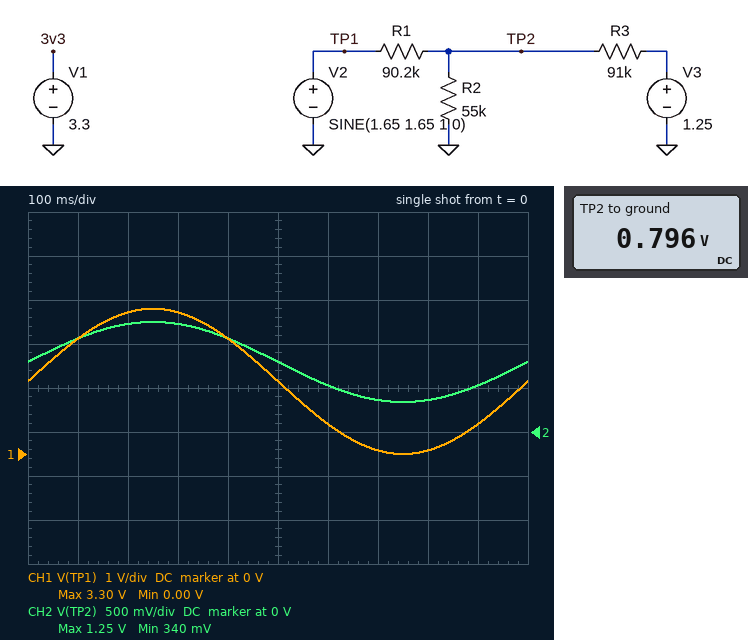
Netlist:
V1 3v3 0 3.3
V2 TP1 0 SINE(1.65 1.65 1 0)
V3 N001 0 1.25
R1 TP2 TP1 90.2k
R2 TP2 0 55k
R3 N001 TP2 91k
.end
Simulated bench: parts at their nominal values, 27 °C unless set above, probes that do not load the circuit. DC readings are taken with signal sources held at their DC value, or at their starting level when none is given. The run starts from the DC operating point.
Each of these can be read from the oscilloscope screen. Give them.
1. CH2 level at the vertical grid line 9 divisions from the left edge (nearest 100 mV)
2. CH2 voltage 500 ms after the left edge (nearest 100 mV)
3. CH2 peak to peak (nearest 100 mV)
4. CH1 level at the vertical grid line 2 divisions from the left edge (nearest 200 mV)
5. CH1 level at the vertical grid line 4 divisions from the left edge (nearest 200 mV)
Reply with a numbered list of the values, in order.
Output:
1. 500 mV
2. 800 mV
3. 900 mV
4. 3.2 V
5. 2.6 V
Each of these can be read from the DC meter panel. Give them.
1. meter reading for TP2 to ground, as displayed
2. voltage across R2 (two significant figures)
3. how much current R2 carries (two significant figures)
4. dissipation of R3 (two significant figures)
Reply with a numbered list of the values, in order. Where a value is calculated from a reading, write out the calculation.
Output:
1. 0.796 V
2. 796 mV = 800 mV
3. (796 mV) / 55 kΩ = 14 µA
4. (1.25 V - 796 mV)^2 / 91 kΩ = 2.3 µW
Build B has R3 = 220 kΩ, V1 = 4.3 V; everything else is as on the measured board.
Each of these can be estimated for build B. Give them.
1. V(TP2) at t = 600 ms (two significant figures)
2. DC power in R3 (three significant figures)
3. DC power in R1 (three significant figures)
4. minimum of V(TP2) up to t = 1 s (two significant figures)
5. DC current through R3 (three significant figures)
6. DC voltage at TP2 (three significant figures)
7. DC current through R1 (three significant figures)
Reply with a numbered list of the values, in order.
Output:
1. 390 mV
2. 1.33 µW
3. 9.82 µW
4. 170 mV
5. 2.46 µA
6. 709 mV
7. 10.4 µA
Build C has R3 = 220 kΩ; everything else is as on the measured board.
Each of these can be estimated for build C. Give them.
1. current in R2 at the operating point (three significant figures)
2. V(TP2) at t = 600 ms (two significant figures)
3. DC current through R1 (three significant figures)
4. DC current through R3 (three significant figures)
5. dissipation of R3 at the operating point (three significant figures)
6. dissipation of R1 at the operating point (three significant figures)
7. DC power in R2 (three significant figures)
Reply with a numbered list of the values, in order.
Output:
1. 12.9 µA
2. 390 mV
3. 10.4 µA
4. 2.46 µA
5. 1.33 µW
6. 9.82 µW
7. 9.14 µW
